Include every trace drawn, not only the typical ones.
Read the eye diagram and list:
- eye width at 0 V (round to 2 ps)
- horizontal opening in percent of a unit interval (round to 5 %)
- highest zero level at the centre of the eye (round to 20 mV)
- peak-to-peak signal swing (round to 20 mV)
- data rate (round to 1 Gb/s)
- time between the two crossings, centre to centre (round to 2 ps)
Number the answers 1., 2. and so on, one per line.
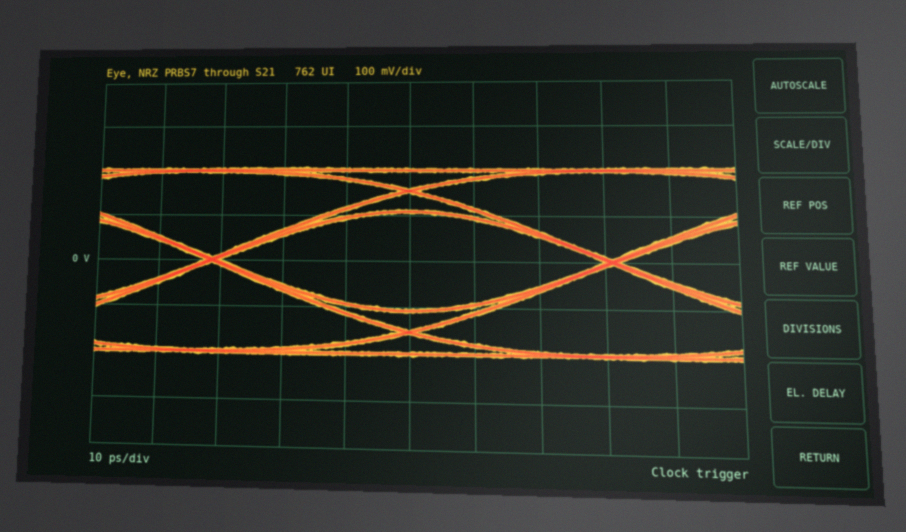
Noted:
1. 60 ps
2. 95 %
3. -100 mV
4. 420 mV
5. 16 Gb/s
6. 62 ps
